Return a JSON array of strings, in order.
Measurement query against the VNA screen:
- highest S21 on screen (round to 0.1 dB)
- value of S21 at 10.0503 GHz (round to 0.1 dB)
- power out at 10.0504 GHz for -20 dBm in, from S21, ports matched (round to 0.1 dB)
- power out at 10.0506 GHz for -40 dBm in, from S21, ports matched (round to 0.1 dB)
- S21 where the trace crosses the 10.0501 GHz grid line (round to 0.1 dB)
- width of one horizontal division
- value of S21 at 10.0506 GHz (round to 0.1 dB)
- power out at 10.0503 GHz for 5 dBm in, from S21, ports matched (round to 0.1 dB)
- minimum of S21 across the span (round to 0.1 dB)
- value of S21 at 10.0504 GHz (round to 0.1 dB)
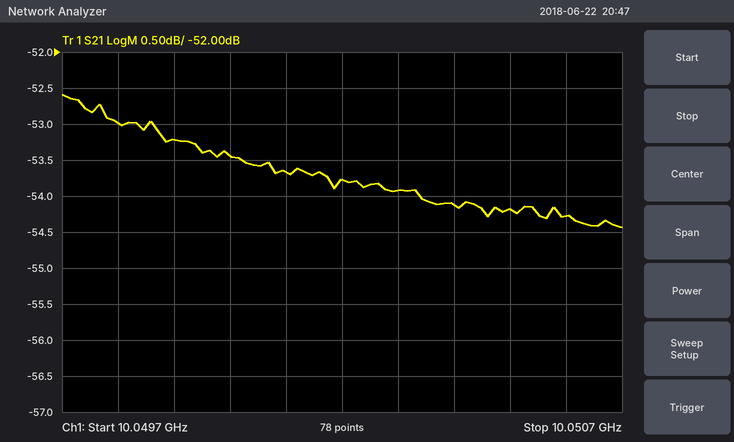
["-52.6 dB", "-53.9 dB", "-74.1 dBm", "-94.3 dBm", "-53.7 dB", "100 kHz", "-54.3 dB", "-48.9 dBm", "-54.4 dB", "-54.1 dB"]
